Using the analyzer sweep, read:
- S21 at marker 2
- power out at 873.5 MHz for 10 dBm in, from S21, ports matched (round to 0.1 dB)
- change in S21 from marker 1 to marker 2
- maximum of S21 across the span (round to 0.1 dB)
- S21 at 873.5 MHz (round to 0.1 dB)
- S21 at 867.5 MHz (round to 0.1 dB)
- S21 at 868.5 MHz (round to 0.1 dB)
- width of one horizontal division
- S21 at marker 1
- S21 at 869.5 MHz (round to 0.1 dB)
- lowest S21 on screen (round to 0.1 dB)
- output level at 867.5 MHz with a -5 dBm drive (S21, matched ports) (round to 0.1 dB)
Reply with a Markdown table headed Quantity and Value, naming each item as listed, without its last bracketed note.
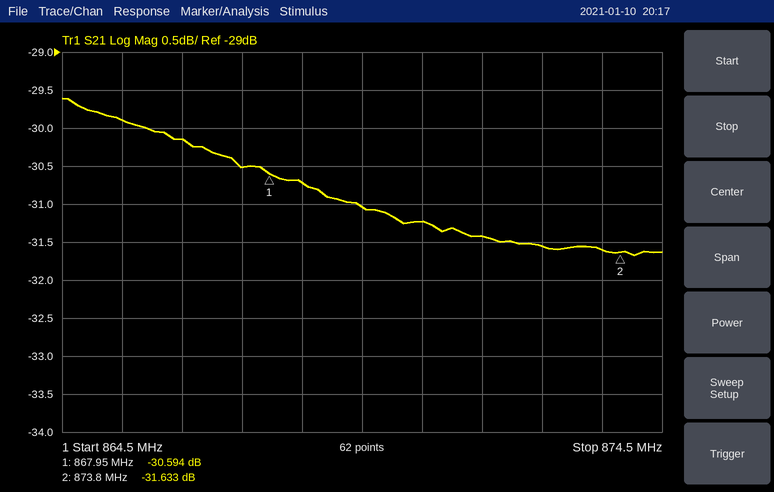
| Quantity | Value |
|---|---|
| S21 at marker 2 | -31.633 dB |
| power out at 873.5 MHz for 10 dBm in, from S21, ports matched | -21.6 dBm |
| change in S21 from marker 1 to marker 2 | -1.039 dB |
| maximum of S21 across the span | -29.6 dB |
| S21 at 873.5 MHz | -31.6 dB |
| S21 at 867.5 MHz | -30.5 dB |
| S21 at 868.5 MHz | -30.7 dB |
| width of one horizontal division | 1 MHz |
| S21 at marker 1 | -30.594 dB |
| S21 at 869.5 MHz | -31.0 dB |
| lowest S21 on screen | -31.7 dB |
| output level at 867.5 MHz with a -5 dBm drive (S21, matched ports) | -35.5 dBm |
